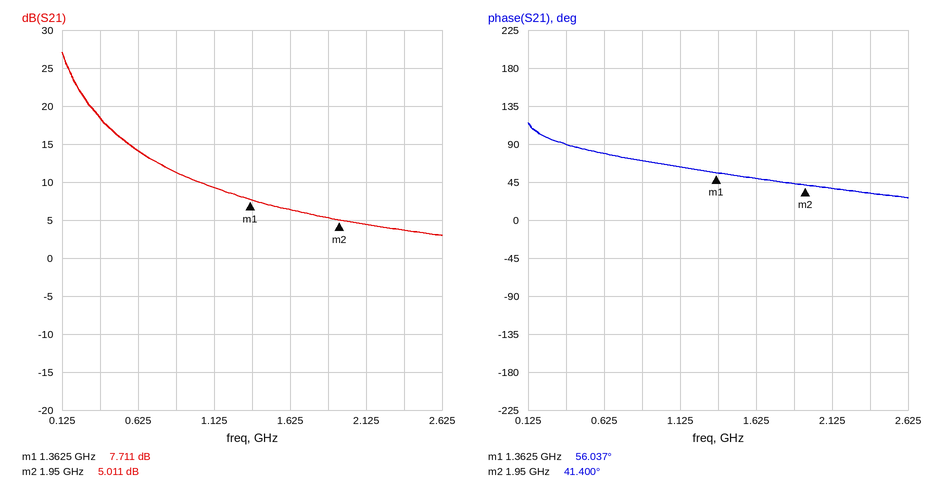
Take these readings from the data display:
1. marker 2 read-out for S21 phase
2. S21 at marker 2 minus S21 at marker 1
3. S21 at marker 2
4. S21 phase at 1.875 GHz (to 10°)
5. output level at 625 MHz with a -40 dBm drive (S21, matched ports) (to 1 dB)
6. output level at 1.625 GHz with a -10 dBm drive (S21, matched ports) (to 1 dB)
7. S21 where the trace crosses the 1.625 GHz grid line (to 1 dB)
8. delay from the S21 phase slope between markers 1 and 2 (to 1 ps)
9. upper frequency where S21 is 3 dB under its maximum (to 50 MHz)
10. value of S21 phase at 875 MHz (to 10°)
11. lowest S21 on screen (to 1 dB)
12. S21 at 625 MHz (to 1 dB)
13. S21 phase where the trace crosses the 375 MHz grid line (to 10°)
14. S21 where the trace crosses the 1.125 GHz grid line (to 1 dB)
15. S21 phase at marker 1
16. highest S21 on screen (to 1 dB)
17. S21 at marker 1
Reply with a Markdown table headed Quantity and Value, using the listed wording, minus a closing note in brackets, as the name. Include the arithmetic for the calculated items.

| Quantity | Value |
|---|---|
| marker 2 read-out for S21 phase | 41.400° |
| S21 at marker 2 minus S21 at marker 1 | 5.011 − (7.711) = -2.700 dB |
| S21 at marker 2 | 5.011 dB |
| S21 phase at 1.875 GHz | 40° |
| output level at 625 MHz with a -40 dBm drive (S21, matched ports) | -40 dBm + (14 dB) = -26 dBm |
| output level at 1.625 GHz with a -10 dBm drive (S21, matched ports) | -10 dBm + (6 dB) = -4 dBm |
| S21 where the trace crosses the 1.625 GHz grid line | 6 dB |
| delay from the S21 phase slope between markers 1 and 2 | −(41.4° − (56.037°))/(360° × 587.5 MHz) ≈ 69 ps |
| upper frequency where S21 is 3 dB under its maximum | 200 MHz |
| value of S21 phase at 875 MHz | 70° |
| lowest S21 on screen | 3 dB |
| S21 at 625 MHz | 14 dB |
| S21 phase where the trace crosses the 375 MHz grid line | 90° |
| S21 where the trace crosses the 1.125 GHz grid line | 9 dB |
| S21 phase at marker 1 | 56.037° |
| highest S21 on screen | 27 dB |
| S21 at marker 1 | 7.711 dB |
